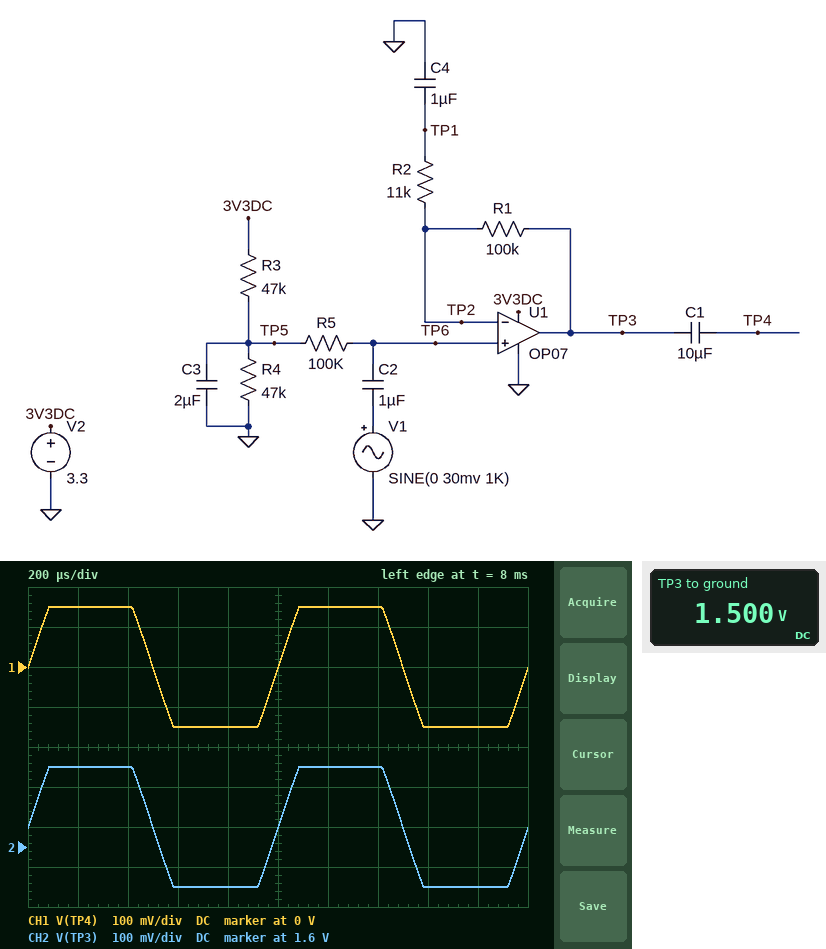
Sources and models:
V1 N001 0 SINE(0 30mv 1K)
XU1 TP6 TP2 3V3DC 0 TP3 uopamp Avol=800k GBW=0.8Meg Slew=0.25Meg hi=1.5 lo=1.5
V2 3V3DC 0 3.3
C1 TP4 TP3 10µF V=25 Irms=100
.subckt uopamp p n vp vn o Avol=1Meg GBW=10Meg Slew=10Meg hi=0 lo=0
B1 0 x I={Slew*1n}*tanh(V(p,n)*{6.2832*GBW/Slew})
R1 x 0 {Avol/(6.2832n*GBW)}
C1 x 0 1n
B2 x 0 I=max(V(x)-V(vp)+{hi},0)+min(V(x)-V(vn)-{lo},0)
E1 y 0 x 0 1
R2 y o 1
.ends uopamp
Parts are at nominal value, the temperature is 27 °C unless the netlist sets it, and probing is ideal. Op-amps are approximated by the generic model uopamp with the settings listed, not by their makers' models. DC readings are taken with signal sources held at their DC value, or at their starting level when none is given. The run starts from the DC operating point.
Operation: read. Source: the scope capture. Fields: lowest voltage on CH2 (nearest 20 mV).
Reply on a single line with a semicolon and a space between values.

1.50 V
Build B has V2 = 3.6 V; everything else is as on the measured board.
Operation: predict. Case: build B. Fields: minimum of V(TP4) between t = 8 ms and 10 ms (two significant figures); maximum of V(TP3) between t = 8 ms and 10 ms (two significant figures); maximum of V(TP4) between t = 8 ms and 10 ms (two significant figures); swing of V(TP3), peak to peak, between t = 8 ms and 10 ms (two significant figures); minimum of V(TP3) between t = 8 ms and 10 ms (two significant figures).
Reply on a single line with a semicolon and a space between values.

-300 mV; 2.1 V; 300 mV; 600 mV; 1.5 V
